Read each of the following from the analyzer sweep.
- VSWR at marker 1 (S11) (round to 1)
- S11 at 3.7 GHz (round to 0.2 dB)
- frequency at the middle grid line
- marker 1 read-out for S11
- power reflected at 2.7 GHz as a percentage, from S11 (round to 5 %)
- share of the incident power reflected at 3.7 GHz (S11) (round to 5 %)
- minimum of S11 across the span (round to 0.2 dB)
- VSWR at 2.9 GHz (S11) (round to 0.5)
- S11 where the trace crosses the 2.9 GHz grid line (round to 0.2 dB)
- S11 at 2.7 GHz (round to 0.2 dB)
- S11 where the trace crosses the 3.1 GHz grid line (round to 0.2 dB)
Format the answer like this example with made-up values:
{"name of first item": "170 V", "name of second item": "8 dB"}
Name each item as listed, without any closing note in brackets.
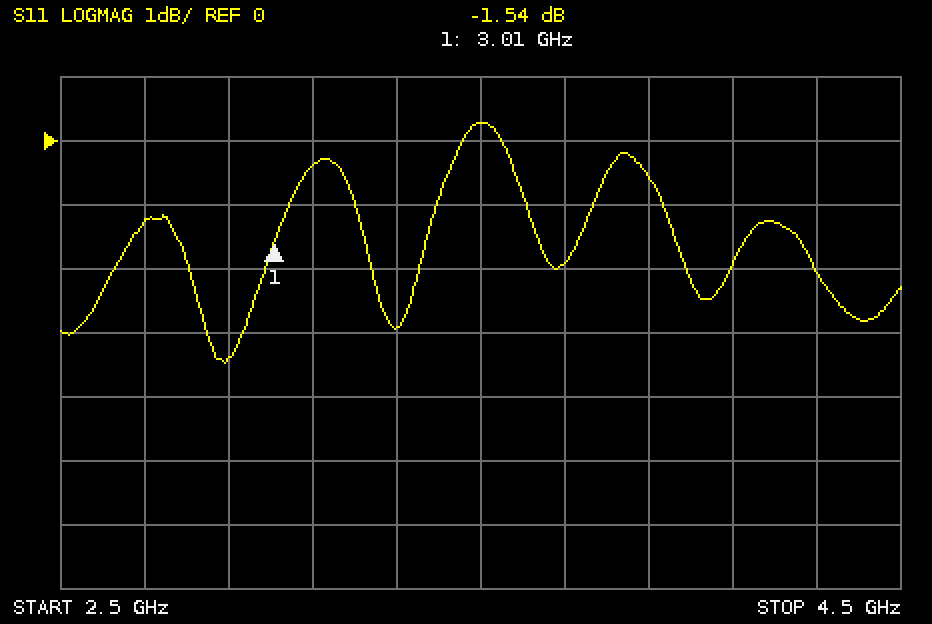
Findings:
{"VSWR at marker 1 (S11)": "11", "S11 at 3.7 GHz": "-2.0 dB", "frequency at the middle grid line": "3.5 GHz", "marker 1 read-out for S11": "-1.54 dB", "power reflected at 2.7 GHz as a percentage, from S11": "75 %", "share of the incident power reflected at 3.7 GHz (S11)": "65 %", "minimum of S11 across the span": "-3.4 dB", "VSWR at 2.9 GHz (S11)": "5.0", "S11 where the trace crosses the 2.9 GHz grid line": "-3.4 dB", "S11 at 2.7 GHz": "-1.2 dB", "S11 where the trace crosses the 3.1 GHz grid line": "-0.4 dB"}
